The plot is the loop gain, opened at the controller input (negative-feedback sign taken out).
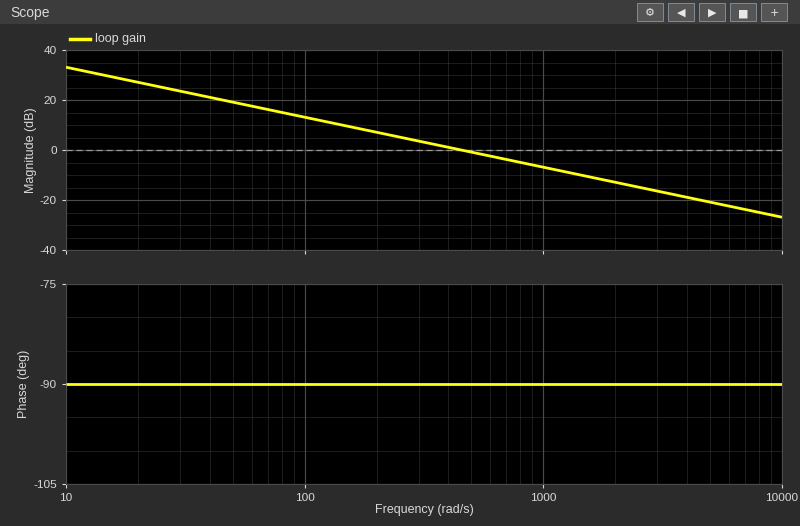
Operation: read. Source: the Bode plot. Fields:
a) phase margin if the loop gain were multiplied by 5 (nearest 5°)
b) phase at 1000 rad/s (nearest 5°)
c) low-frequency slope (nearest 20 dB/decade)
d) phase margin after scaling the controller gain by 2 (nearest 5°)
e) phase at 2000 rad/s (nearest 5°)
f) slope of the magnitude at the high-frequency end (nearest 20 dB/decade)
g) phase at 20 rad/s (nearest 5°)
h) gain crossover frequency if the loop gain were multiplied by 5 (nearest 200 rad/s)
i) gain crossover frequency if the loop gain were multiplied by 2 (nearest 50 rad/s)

90°
-90°
-20 dB/decade
90°
-90°
-20 dB/decade
-90°
2200 rad/s
900 rad/s
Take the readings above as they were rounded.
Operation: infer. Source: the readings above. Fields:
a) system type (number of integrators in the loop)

1
